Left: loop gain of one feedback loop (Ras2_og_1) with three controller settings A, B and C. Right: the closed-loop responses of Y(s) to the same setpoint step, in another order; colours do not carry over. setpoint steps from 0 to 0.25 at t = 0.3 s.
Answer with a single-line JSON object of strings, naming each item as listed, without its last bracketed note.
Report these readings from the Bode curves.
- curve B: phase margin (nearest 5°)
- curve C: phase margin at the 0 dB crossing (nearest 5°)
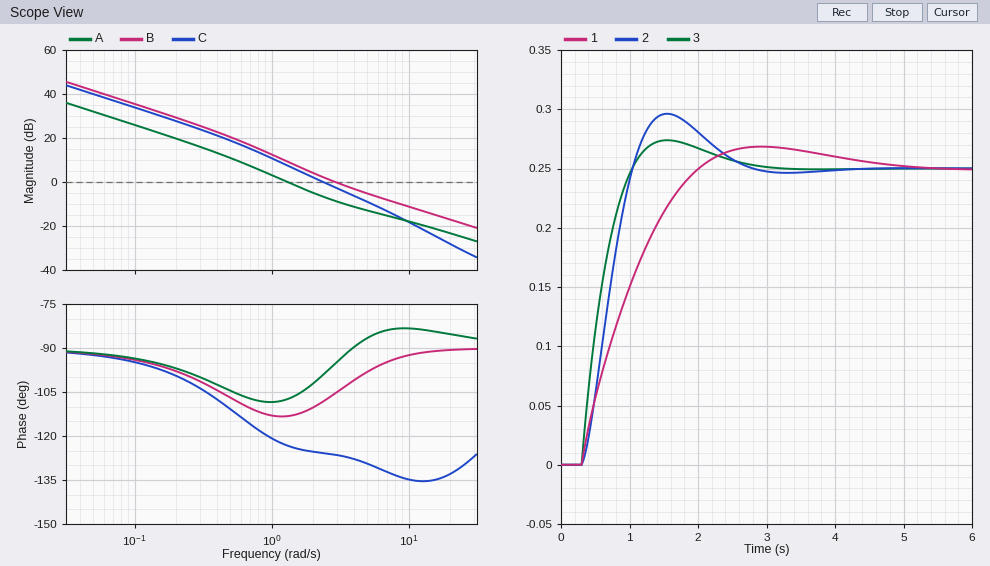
{"curve B: phase margin": "75°", "curve C: phase margin at the 0 dB crossing": "55°"}
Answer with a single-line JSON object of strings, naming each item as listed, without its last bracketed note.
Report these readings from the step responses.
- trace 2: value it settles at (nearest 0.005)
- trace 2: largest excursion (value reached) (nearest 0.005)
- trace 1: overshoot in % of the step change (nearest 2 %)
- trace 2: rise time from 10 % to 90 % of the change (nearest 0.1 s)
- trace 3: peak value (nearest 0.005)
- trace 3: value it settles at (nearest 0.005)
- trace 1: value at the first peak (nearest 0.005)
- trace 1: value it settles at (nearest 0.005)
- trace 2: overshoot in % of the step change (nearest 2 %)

{"trace 2: value it settles at": "0.250", "trace 2: largest excursion (value reached)": "0.295", "trace 1: overshoot in % of the step change": "8 %", "trace 2: rise time from 10 % to 90 % of the change": "0.5 s", "trace 3: peak value": "0.275", "trace 3: value it settles at": "0.250", "trace 1: value at the first peak": "0.270", "trace 1: value it settles at": "0.250", "trace 2: overshoot in % of the step change": "18 %"}
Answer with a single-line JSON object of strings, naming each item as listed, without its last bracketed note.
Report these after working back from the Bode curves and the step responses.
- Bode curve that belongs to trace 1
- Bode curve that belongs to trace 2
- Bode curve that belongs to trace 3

{"Bode curve that belongs to trace 1": "A", "Bode curve that belongs to trace 2": "C", "Bode curve that belongs to trace 3": "B"}
